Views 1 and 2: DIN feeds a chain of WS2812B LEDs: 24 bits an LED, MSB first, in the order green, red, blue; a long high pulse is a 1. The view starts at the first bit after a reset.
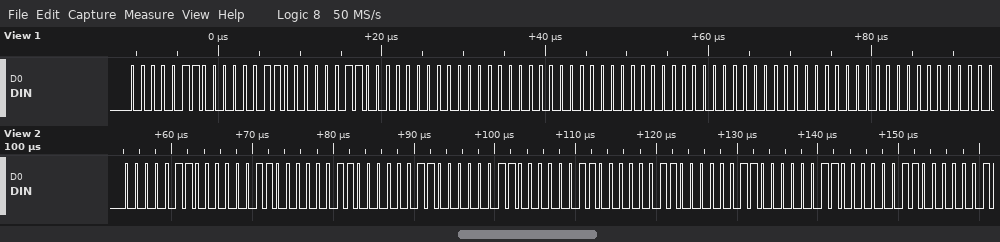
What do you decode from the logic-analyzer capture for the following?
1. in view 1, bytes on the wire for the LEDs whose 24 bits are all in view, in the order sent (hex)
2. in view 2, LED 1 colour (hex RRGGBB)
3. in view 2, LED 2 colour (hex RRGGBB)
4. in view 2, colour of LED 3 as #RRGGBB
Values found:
06 06 06 00 00 00 00 00 00
#060606
#060606
#060606
